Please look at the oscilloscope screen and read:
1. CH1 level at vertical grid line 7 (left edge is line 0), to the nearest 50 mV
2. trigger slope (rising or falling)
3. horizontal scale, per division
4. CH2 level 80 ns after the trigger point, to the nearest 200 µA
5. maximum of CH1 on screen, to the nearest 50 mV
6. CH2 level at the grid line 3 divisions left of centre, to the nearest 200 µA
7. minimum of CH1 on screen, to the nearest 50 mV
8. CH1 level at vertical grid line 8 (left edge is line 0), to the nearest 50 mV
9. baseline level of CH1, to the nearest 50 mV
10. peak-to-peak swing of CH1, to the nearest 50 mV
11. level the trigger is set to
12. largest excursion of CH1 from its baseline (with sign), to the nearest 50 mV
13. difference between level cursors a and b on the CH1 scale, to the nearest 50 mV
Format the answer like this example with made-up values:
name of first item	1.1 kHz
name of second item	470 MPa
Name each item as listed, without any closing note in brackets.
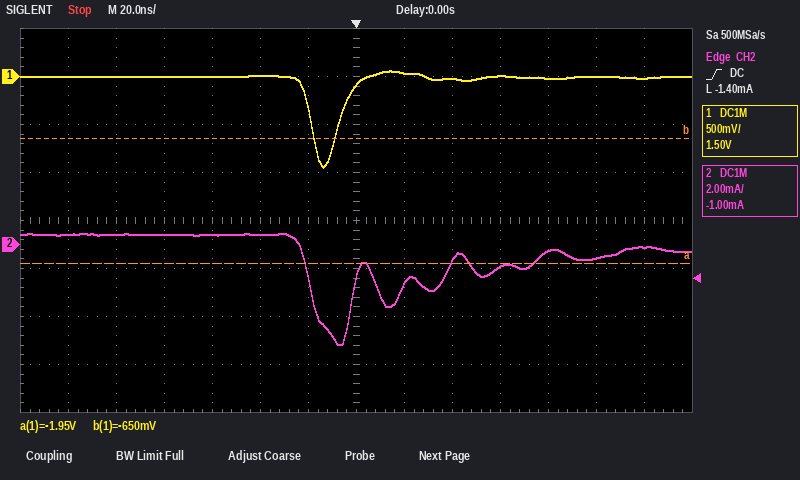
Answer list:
CH1 level at vertical grid line 7 (left edge is line 0), to the nearest 50 mV	-100 mV
trigger slope	rising
horizontal scale, per division	20 ns
CH2 level 80 ns after the trigger point, to the nearest 200 µA	-200 µA
maximum of CH1 on screen, to the nearest 50 mV	50 mV
CH2 level at the grid line 3 divisions left of centre, to the nearest 200 µA	400 µA
minimum of CH1 on screen, to the nearest 50 mV	-950 mV
CH1 level at vertical grid line 8 (left edge is line 0), to the nearest 50 mV	50 mV
baseline level of CH1, to the nearest 50 mV	0 mV
peak-to-peak swing of CH1, to the nearest 50 mV	1.00 V
level the trigger is set to	-1.40 mA
largest excursion of CH1 from its baseline (with sign), to the nearest 50 mV	-950 mV
difference between level cursors a and b on the CH1 scale, to the nearest 50 mV	1.30 V
